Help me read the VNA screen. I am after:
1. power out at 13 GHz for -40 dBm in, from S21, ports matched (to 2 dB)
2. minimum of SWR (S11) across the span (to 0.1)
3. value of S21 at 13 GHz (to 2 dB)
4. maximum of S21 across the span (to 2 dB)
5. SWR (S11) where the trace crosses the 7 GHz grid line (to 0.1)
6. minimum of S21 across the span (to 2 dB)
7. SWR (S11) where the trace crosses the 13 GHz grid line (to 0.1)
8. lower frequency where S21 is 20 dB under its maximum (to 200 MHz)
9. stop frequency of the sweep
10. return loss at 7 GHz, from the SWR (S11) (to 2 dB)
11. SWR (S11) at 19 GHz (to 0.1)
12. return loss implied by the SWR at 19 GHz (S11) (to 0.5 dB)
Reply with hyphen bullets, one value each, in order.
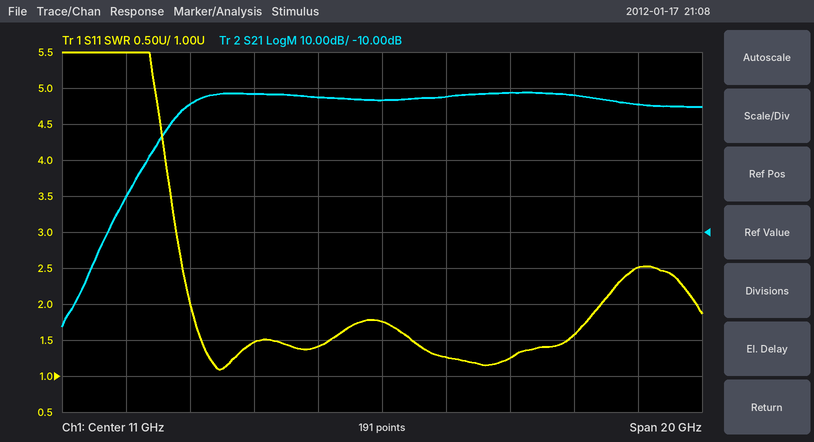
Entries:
- -12 dBm
- 1.1
- 28 dB
- 28 dB
- 1.5
- -36 dB
- 1.3
- 3.6 GHz
- 21 GHz
- 14 dB
- 2.5
- 7.5 dB
